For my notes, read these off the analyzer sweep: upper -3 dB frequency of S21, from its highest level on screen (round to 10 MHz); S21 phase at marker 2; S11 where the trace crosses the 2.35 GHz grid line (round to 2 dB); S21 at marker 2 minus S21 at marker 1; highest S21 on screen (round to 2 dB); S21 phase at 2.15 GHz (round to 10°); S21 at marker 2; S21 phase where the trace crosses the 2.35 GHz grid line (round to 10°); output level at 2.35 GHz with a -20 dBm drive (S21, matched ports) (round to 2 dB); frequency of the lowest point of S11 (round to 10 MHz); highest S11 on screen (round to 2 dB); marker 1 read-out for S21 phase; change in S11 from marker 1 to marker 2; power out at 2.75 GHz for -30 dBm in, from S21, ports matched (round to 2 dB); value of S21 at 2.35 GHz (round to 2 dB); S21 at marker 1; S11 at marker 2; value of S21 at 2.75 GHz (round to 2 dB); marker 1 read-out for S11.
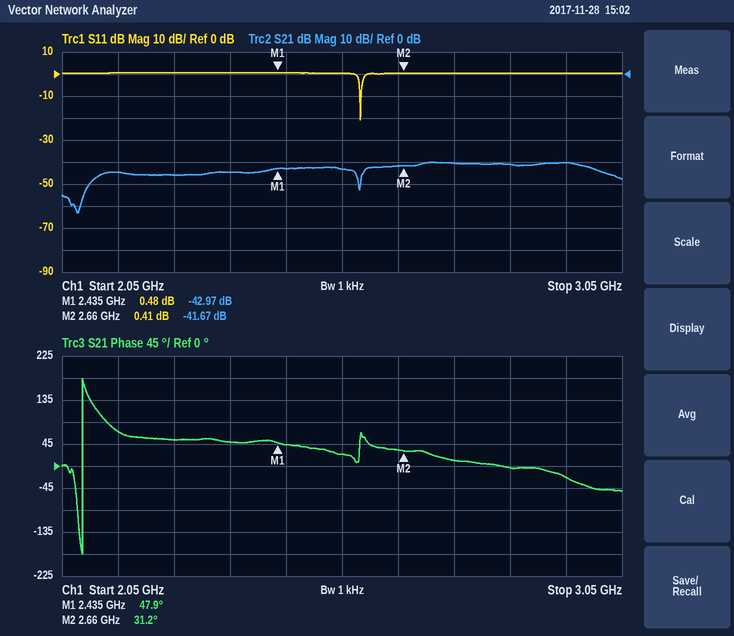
3.00 GHz
31.2°
0 dB
1.30 dB
-40 dB
70°
-41.67 dB
50°
-64 dBm
2.58 GHz
0 dB
47.9°
-0.07 dB
-70 dBm
-44 dB
-42.97 dB
0.41 dB
-40 dB
0.48 dB
